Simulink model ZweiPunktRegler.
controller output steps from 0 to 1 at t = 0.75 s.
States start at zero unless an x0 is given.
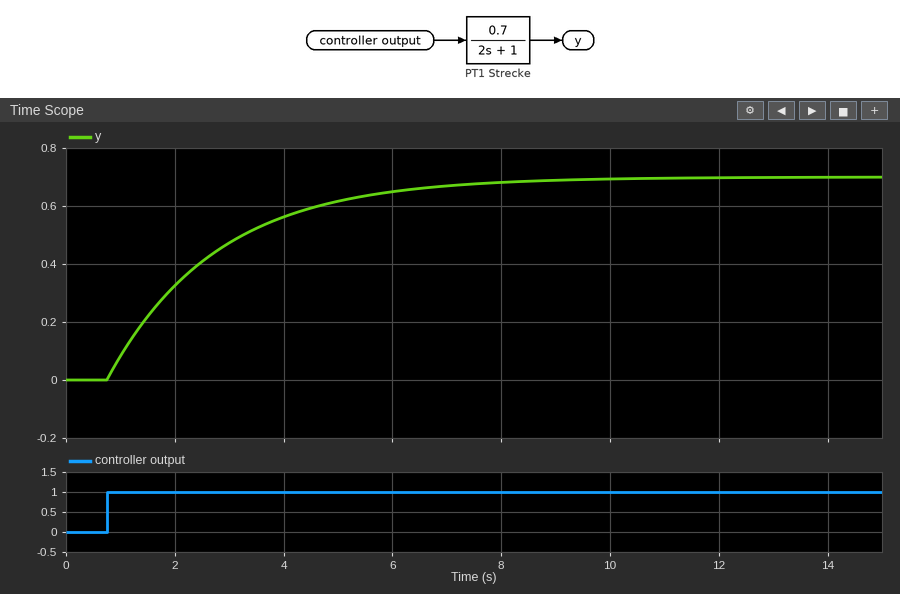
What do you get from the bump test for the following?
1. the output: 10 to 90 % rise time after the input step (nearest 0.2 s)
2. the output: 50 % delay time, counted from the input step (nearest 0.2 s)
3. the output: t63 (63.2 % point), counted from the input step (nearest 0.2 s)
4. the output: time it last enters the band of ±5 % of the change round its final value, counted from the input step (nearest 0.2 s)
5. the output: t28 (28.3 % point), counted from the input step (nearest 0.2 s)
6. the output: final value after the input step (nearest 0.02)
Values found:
4.4 s
1.4 s
2.0 s
6.0 s
0.6 s
0.70
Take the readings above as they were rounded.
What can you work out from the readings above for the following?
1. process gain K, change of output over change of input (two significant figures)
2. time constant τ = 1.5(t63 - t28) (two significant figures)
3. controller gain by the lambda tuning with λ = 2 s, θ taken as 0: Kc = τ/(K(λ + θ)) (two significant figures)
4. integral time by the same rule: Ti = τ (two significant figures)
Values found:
0.70
2.1 s
1.5
2.1 s
